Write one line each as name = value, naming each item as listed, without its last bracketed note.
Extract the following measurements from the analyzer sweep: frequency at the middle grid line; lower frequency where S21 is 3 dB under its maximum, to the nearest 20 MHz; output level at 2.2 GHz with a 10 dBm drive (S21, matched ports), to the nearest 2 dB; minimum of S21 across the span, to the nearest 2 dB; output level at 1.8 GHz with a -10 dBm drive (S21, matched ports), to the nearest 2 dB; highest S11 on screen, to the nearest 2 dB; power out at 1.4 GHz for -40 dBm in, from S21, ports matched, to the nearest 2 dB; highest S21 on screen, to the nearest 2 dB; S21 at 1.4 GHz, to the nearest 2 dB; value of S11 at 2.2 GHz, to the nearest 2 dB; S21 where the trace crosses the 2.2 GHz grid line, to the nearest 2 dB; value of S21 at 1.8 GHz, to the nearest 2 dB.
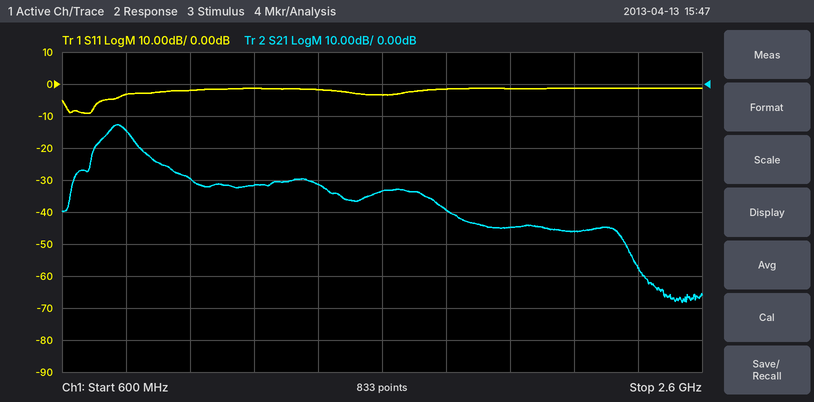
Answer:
frequency at the middle grid line = 1.6 GHz
lower frequency where S21 is 3 dB under its maximum, to the nearest 20 MHz = 740 MHz
output level at 2.2 GHz with a 10 dBm drive (S21, matched ports), to the nearest 2 dB = -36 dBm
minimum of S21 across the span, to the nearest 2 dB = -68 dB
output level at 1.8 GHz with a -10 dBm drive (S21, matched ports), to the nearest 2 dB = -50 dBm
highest S11 on screen, to the nearest 2 dB = -2 dB
power out at 1.4 GHz for -40 dBm in, from S21, ports matched, to the nearest 2 dB = -72 dBm
highest S21 on screen, to the nearest 2 dB = -12 dB
S21 at 1.4 GHz, to the nearest 2 dB = -32 dB
value of S11 at 2.2 GHz, to the nearest 2 dB = -2 dB
S21 where the trace crosses the 2.2 GHz grid line, to the nearest 2 dB = -46 dB
value of S21 at 1.8 GHz, to the nearest 2 dB = -40 dB
